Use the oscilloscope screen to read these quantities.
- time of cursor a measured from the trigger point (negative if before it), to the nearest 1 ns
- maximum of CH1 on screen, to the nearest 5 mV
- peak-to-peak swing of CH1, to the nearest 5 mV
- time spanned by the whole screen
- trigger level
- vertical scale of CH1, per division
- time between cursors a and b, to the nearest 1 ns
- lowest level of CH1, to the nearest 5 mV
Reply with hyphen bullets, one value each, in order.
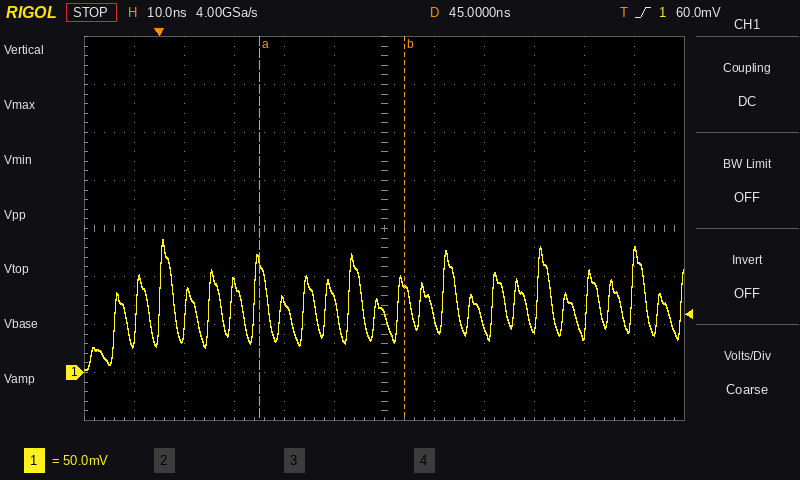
- +20 ns
- 140 mV
- 135 mV
- 120 ns
- 60.0 mV
- 50 mV
- 29 ns
- 5 mV
